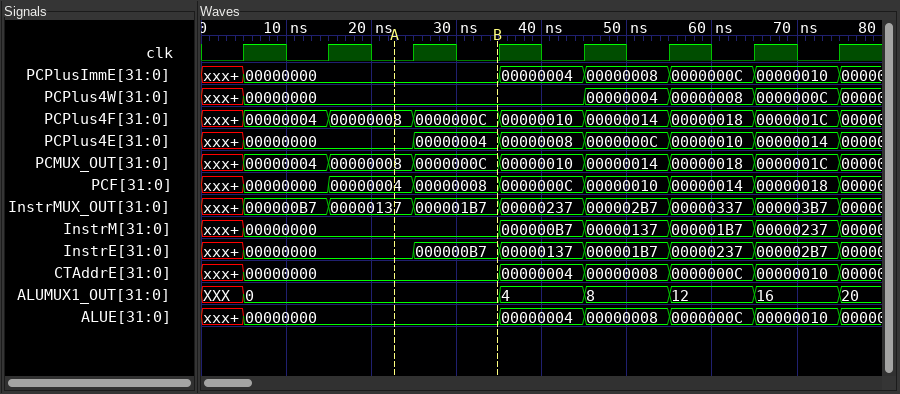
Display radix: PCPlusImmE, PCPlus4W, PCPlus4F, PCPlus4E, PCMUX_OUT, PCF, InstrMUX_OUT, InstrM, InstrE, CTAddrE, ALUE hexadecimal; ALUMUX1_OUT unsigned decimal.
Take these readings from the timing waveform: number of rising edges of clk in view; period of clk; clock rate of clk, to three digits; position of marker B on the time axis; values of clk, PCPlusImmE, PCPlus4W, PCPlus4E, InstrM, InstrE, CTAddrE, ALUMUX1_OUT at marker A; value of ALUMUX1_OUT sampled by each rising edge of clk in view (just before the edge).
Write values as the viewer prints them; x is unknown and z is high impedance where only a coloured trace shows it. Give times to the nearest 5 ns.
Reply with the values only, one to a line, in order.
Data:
8
10 ns
100 MHz
35 ns
clk=0, PCPlusImmE=00000000, PCPlus4W=00000000, PCPlus4E=00000000, InstrM=00000000, InstrE=00000000, CTAddrE=00000000, ALUMUX1_OUT=0
XXX, 0, 0, 0, 4, 8, 12, 16
